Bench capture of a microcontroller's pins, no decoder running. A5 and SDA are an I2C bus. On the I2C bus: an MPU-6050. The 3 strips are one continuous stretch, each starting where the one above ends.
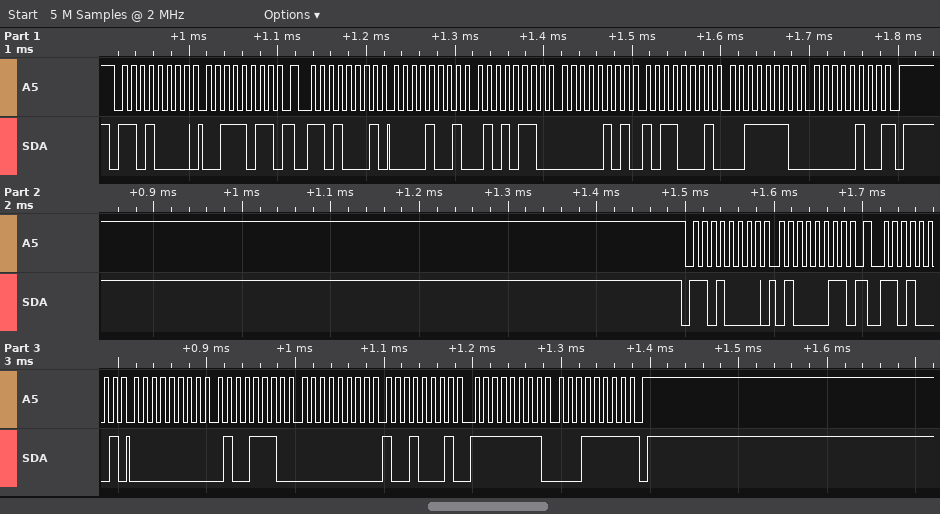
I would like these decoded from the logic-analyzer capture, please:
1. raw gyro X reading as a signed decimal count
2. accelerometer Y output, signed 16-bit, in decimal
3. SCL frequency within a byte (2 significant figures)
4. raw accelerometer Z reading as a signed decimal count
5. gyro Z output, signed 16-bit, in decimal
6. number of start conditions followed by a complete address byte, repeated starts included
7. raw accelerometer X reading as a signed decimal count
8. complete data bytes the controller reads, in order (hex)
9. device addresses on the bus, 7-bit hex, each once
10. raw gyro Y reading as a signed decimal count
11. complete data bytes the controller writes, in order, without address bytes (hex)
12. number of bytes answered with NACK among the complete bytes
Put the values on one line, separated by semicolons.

78; 1457; 100 kHz; 15876; -225; 4; 2390; 09 56 05 B1 3E 04 00 4E 00 91 FF 1F; 0x68; 145; 3B 43; 2
